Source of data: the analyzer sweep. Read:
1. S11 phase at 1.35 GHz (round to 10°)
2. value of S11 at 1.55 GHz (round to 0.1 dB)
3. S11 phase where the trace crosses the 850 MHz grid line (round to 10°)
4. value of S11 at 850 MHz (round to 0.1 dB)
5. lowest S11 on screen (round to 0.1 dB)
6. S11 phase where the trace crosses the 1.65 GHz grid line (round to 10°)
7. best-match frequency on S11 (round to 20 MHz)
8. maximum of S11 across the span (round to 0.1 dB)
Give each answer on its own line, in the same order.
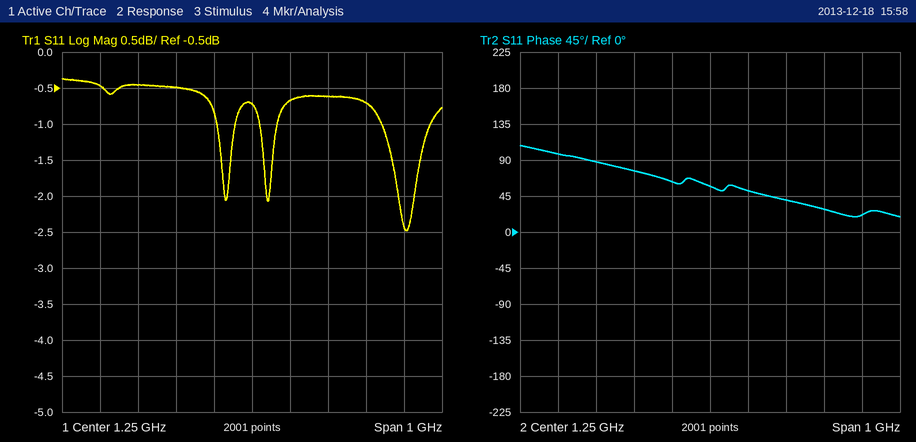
50°
-0.7 dB
100°
-0.5 dB
-2.5 dB
20°
1.66 GHz
-0.4 dB
